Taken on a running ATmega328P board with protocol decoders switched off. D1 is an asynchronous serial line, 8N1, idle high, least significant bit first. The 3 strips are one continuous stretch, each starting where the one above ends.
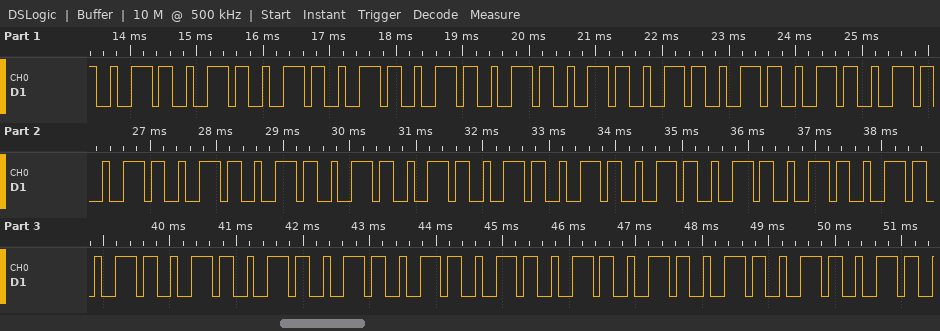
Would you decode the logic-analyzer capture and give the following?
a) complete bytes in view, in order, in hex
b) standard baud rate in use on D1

72 72 72 72 72 72 72 72 72 72 72 72 72 72 72 72 72 72 72 72 72 72 72 72 72 72 72 72 72 72 72 72 72
9600 baud
